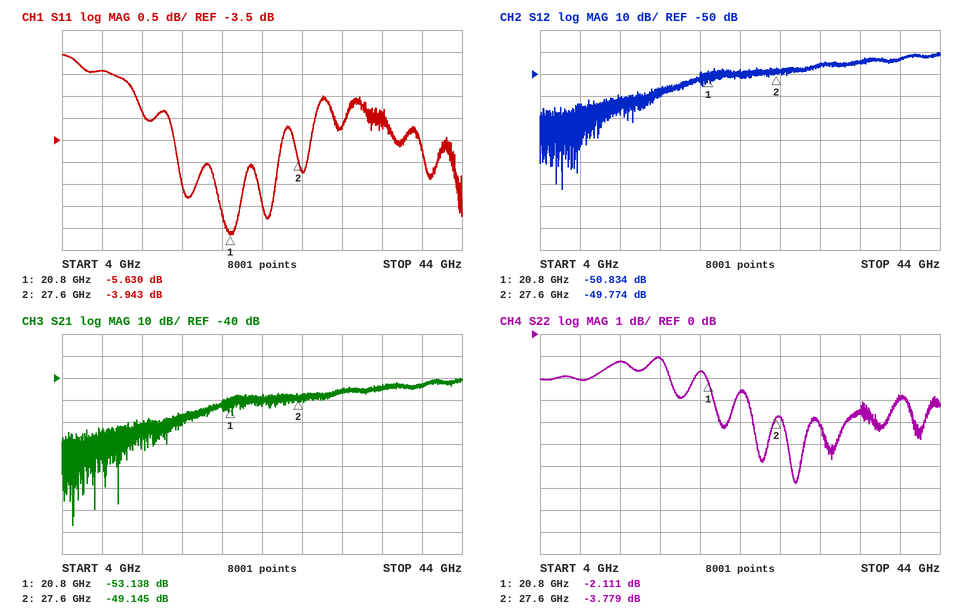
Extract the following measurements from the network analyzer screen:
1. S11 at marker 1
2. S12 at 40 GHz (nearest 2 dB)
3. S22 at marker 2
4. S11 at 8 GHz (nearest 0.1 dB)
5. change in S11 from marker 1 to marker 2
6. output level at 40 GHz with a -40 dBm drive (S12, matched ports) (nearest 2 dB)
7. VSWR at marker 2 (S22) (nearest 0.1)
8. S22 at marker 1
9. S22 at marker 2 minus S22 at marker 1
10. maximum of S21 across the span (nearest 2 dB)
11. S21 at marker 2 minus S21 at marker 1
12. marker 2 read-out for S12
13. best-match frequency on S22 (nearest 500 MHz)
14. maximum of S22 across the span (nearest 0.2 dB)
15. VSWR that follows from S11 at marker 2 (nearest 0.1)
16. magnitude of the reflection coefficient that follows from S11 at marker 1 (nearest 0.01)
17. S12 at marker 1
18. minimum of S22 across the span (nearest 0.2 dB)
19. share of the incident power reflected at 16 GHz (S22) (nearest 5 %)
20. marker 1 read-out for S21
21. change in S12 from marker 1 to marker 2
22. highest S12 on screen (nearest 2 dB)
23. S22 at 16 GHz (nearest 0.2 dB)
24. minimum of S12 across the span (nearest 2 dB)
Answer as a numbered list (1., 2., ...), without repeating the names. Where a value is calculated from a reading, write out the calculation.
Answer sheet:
1. -5.630 dB
2. -44 dB
3. -3.779 dB
4. -1.9 dB
5. -3.943 − (-5.63) = 1.687 dB
6. -40 dBm + (-44 dB) = -84 dBm
7. (1 + 0.6472)/(1 − 0.6472) ≈ 4.7
8. -2.111 dB
9. -3.779 − (-2.111) = -1.668 dB
10. -40 dB
11. -49.145 − (-53.138) = 3.993 dB
12. -49.774 dB
13. 29.5 GHz
14. -1.0 dB
15. (1 + 0.6351)/(1 − 0.6351) ≈ 4.5
16. 10^(-5.63/20) ≈ 0.52
17. -50.834 dB
18. -6.8 dB
19. 10^(-1/10) ≈ 79.4 %, so 80 % to the nearest 5 %
20. -53.138 dB
21. -49.774 − (-50.834) = 1.060 dB
22. -40 dB
23. -1.0 dB
24. -102 dB
